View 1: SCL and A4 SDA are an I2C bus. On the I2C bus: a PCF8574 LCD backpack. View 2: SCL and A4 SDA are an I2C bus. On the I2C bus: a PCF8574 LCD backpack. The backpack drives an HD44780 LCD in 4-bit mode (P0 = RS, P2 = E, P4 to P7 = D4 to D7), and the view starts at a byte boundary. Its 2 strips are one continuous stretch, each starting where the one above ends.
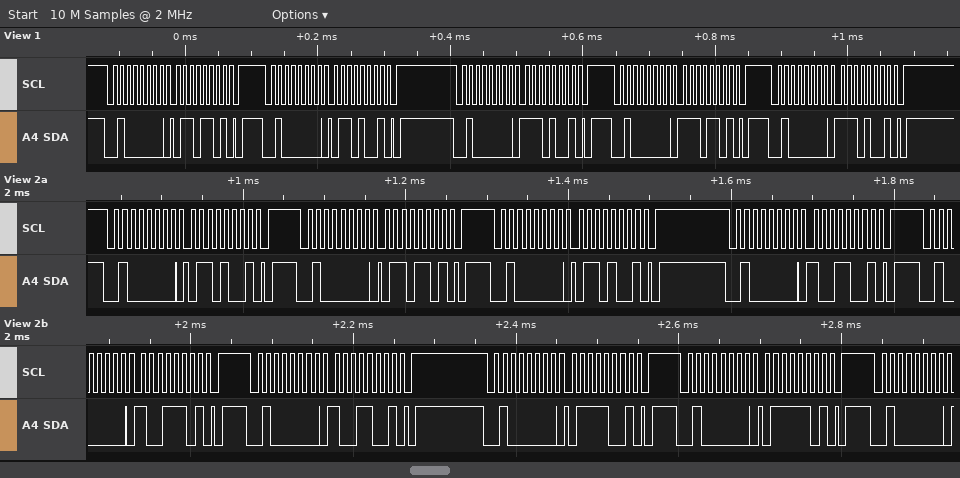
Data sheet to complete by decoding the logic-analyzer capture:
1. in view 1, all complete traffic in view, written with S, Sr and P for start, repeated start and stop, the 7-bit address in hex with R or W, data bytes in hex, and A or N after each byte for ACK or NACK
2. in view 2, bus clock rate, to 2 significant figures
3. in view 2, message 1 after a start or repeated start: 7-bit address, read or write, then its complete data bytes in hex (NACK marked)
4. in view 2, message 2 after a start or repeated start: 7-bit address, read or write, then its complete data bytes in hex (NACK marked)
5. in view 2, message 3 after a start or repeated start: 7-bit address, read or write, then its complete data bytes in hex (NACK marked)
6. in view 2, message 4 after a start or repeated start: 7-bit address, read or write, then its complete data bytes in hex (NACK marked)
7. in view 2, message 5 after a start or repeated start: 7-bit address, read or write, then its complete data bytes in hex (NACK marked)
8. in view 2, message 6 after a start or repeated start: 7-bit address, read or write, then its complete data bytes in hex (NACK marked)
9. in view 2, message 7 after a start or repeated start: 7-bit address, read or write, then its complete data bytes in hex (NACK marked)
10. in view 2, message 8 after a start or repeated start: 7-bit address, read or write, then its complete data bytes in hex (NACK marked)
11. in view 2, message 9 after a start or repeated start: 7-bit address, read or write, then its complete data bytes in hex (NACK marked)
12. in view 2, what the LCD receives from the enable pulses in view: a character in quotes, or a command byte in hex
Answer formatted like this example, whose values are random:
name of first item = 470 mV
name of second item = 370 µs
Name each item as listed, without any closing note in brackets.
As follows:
in view 1, all complete traffic in view, written with S, Sr and P for start, repeated start and stop, the 7-bit address in hex with R or W, data bytes in hex, and A or N after each byte for ACK or NACK = S 20W A 6D A P S 20W A 69 A P S 20W A E9 A P S 20W A ED A P S 20W A E9 A P
in view 2, bus clock rate, to 2 significant figures = 100 kHz
in view 2, message 1 after a start or repeated start: 7-bit address, read or write, then its complete data bytes in hex = 0x20 write: 69
in view 2, message 2 after a start or repeated start: 7-bit address, read or write, then its complete data bytes in hex = 0x20 write: 6D
in view 2, message 3 after a start or repeated start: 7-bit address, read or write, then its complete data bytes in hex = 0x20 write: 69
in view 2, message 4 after a start or repeated start: 7-bit address, read or write, then its complete data bytes in hex = 0x20 write: 99
in view 2, message 5 after a start or repeated start: 7-bit address, read or write, then its complete data bytes in hex = 0x20 write: 9D
in view 2, message 6 after a start or repeated start: 7-bit address, read or write, then its complete data bytes in hex = 0x20 write: 99
in view 2, message 7 after a start or repeated start: 7-bit address, read or write, then its complete data bytes in hex = 0x20 write: 79
in view 2, message 8 after a start or repeated start: 7-bit address, read or write, then its complete data bytes in hex = 0x20 write: 7D
in view 2, message 9 after a start or repeated start: 7-bit address, read or write, then its complete data bytes in hex = 0x20 write
in view 2, what the LCD receives from the enable pulses in view: a character in quotes, or a command byte in hex = 'i'
